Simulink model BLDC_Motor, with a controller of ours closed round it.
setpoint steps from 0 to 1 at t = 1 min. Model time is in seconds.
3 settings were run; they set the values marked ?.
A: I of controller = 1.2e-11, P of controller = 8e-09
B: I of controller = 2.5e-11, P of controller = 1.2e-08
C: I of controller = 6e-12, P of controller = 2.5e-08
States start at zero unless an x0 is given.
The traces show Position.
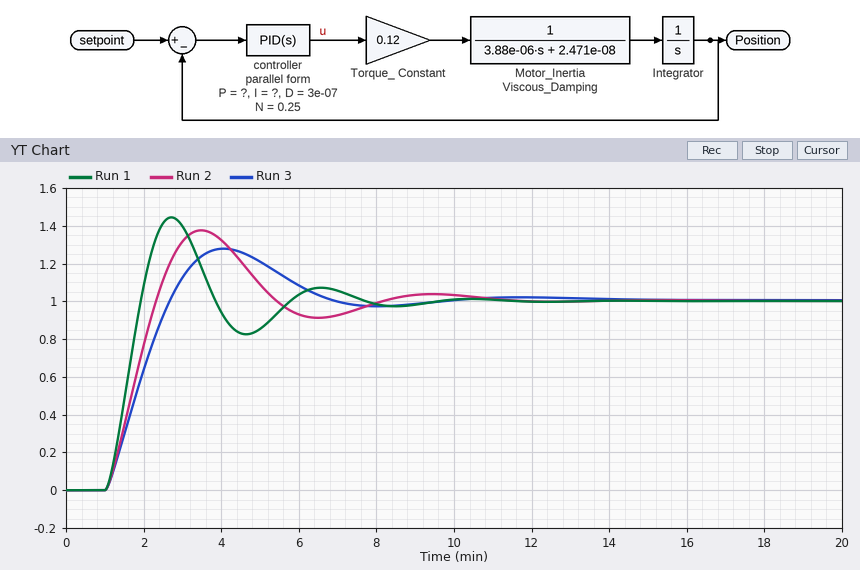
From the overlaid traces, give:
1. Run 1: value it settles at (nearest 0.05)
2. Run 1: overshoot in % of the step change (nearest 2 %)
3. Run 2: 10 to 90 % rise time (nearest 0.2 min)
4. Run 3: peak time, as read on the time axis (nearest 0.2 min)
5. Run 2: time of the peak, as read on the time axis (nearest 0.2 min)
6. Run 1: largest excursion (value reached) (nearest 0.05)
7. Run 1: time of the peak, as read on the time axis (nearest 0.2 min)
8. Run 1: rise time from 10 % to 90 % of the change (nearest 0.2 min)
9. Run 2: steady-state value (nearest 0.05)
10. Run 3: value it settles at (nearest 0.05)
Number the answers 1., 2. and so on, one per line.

1. 1.00
2. 44 %
3. 1.0 min
4. 4.0 min
5. 3.4 min
6. 1.45
7. 2.8 min
8. 0.6 min
9. 1.00
10. 1.00
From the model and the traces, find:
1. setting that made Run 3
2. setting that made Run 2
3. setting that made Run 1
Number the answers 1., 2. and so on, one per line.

1. A
2. B
3. C
